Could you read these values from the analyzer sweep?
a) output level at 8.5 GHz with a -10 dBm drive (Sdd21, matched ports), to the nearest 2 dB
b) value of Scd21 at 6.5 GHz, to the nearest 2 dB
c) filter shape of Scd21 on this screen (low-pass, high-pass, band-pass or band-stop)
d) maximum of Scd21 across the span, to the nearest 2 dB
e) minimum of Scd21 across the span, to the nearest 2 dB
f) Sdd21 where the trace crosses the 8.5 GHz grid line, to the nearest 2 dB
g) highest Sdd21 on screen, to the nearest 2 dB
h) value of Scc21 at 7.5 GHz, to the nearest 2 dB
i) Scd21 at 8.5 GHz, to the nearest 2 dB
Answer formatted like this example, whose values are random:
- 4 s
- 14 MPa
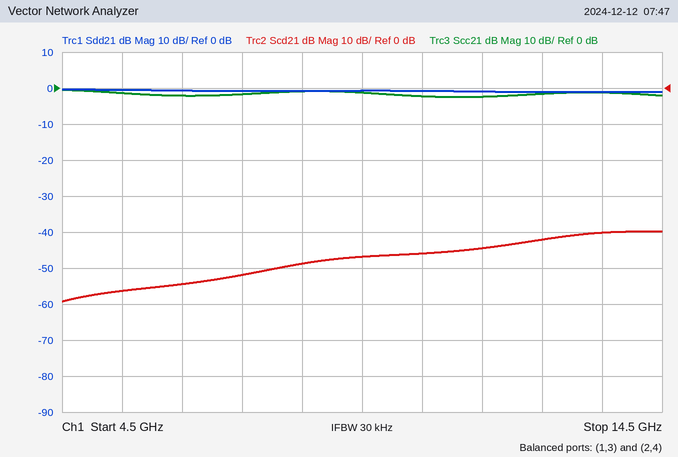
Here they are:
- -10 dBm
- -54 dB
- high-pass
- -40 dB
- -60 dB
- 0 dB
- 0 dB
- -2 dB
- -48 dB
